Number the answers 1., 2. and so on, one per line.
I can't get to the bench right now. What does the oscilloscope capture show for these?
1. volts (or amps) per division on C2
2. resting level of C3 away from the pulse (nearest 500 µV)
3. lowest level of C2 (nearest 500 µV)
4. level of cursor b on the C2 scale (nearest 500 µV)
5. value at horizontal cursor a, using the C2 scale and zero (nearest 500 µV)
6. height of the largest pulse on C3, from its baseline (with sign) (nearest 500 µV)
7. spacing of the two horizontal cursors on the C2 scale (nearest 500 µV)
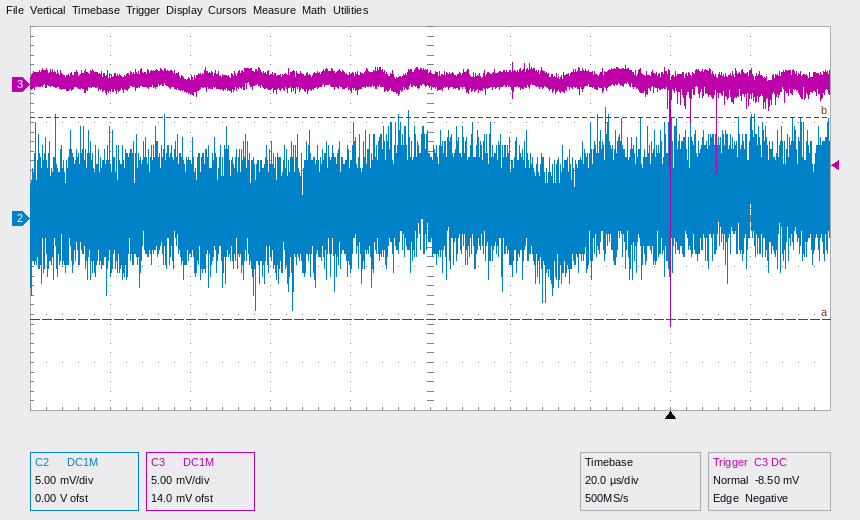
1. 5 mV
2. 500 µV
3. -9.5 mV
4. 10.5 mV
5. -10.5 mV
6. -25.5 mV
7. 21.0 mV
